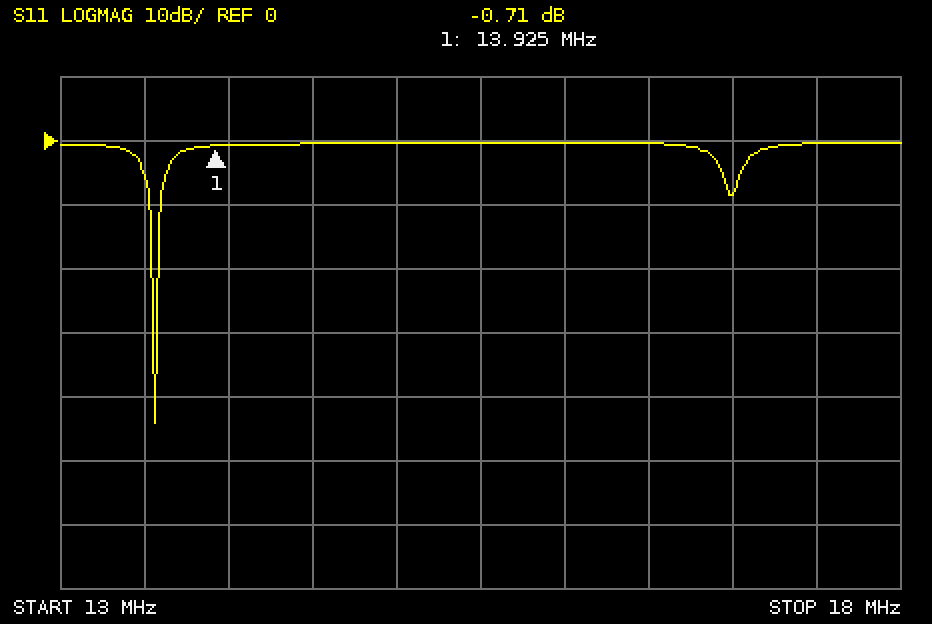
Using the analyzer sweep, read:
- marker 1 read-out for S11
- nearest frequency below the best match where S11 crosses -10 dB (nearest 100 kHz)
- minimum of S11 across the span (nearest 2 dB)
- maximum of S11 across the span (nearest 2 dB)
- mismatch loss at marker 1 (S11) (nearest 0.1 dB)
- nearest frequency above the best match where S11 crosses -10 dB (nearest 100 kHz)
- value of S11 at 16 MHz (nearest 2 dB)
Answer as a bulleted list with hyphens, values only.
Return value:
- -0.71 dB
- 13.5 MHz
- -44 dB
- 0 dB
- 8.2 dB
- 13.6 MHz
- 0 dB
